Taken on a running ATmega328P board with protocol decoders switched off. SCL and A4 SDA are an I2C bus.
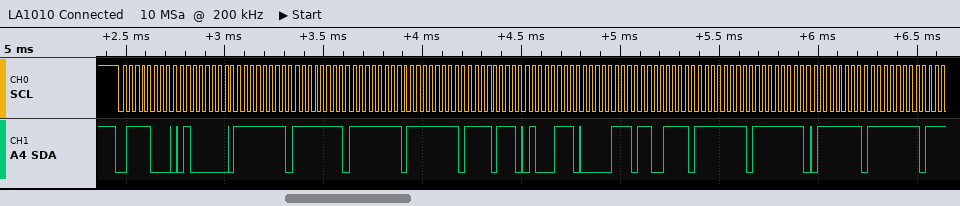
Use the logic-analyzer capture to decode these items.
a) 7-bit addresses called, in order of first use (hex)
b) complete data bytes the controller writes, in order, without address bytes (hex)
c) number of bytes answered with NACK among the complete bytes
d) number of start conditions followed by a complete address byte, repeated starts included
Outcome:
0x3C
40 FF FF FF FF F7 47 07 CF FF FF 7F FF
0
1
